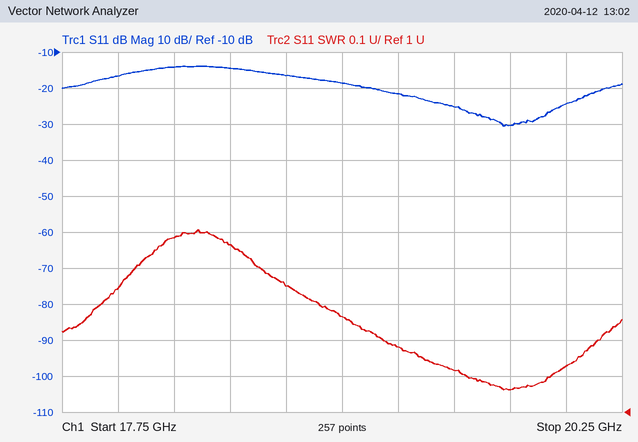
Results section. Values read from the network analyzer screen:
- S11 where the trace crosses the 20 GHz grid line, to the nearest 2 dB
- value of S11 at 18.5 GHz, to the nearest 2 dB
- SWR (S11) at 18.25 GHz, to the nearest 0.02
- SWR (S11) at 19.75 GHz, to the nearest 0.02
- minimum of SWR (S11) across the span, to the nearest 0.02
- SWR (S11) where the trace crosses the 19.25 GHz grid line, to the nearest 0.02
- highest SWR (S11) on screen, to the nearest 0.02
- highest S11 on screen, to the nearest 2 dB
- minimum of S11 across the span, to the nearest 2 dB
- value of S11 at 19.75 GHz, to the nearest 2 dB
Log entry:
-24 dB
-14 dB
1.48
1.06
1.06
1.18
1.50
-14 dB
-30 dB
-30 dB
